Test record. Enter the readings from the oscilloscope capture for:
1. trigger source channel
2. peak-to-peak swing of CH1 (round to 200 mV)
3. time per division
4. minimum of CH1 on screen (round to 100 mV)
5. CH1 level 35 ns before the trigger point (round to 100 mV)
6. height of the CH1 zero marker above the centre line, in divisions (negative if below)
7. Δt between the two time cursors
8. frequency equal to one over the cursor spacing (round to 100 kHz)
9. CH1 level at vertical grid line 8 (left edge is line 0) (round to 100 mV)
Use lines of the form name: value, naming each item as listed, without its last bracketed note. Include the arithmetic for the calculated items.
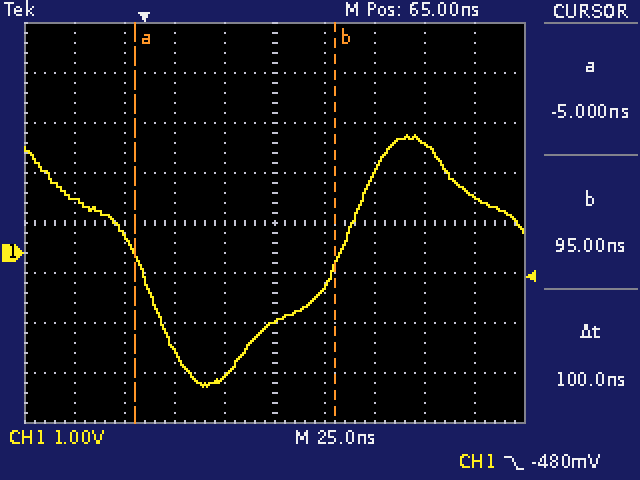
trigger source channel: CH1
peak-to-peak swing of CH1: 5.0 V
time per division: 25 ns
minimum of CH1 on screen: -2.7 V
CH1 level 35 ns before the trigger point: 1.1 V
height of the CH1 zero marker above the centre line, in divisions: -0.6 div
Δt between the two time cursors: 100 ns
frequency equal to one over the cursor spacing: 1 / 100 ns ≈ 10.0 MHz
CH1 level at vertical grid line 8 (left edge is line 0): 2.2 V
